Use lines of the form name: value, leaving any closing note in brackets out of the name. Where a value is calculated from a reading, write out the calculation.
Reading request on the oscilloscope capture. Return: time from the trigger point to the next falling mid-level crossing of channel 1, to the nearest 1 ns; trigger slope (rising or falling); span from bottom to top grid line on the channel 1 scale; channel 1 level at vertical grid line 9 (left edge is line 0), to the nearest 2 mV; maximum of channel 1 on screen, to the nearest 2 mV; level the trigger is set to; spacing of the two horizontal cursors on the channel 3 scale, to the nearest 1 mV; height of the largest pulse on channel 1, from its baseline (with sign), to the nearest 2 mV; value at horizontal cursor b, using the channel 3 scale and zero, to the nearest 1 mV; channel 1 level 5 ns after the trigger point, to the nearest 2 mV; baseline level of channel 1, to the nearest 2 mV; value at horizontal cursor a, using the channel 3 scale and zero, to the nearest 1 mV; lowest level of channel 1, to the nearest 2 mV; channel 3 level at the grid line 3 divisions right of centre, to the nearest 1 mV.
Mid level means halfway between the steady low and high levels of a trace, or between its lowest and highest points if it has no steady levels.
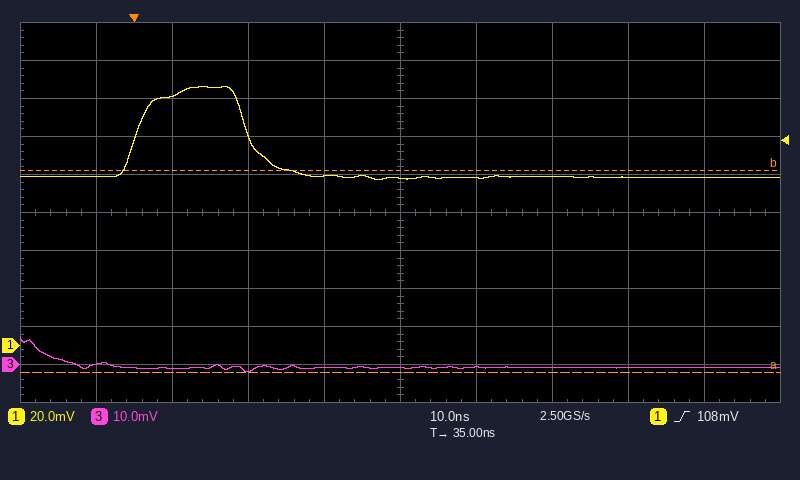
time from the trigger point to the next falling mid-level crossing of channel 1, to the nearest 1 ns: 15 ns
trigger slope: rising
span from bottom to top grid line on the channel 1 scale: 200 mV
channel 1 level at vertical grid line 9 (left edge is line 0), to the nearest 2 mV: 88 mV
maximum of channel 1 on screen, to the nearest 2 mV: 136 mV
level the trigger is set to: 108 mV
spacing of the two horizontal cursors on the channel 3 scale, to the nearest 1 mV: 53 mV
height of the largest pulse on channel 1, from its baseline (with sign), to the nearest 2 mV: 136 mV − (88 mV) = +48 mV
value at horizontal cursor b, using the channel 3 scale and zero, to the nearest 1 mV: 51 mV
channel 1 level 5 ns after the trigger point, to the nearest 2 mV: 132 mV
baseline level of channel 1, to the nearest 2 mV: 88 mV
value at horizontal cursor a, using the channel 3 scale and zero, to the nearest 1 mV: -2 mV
lowest level of channel 1, to the nearest 2 mV: 88 mV
channel 3 level at the grid line 3 divisions right of centre, to the nearest 1 mV: -1 mV
